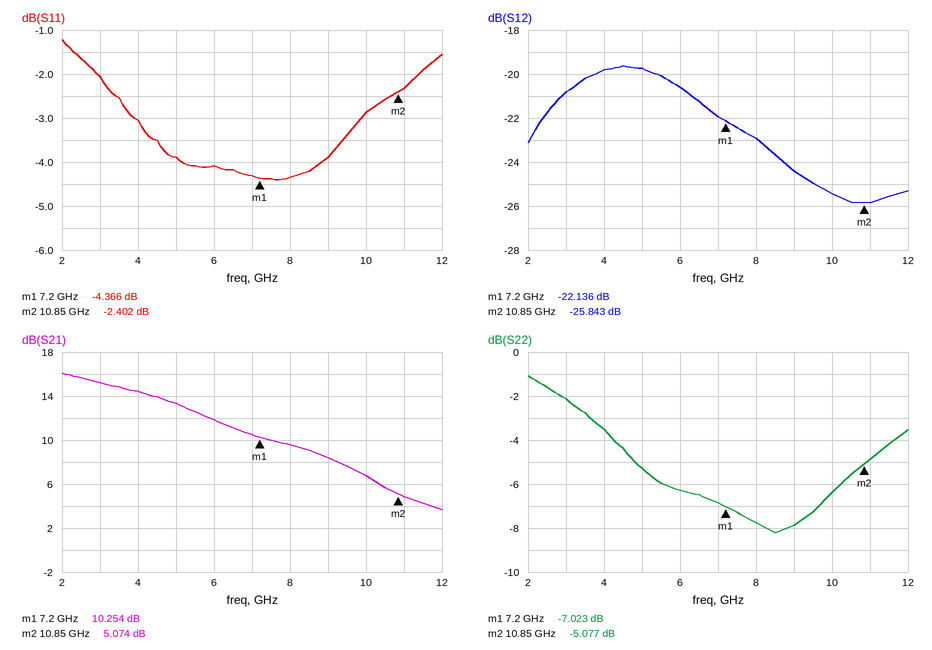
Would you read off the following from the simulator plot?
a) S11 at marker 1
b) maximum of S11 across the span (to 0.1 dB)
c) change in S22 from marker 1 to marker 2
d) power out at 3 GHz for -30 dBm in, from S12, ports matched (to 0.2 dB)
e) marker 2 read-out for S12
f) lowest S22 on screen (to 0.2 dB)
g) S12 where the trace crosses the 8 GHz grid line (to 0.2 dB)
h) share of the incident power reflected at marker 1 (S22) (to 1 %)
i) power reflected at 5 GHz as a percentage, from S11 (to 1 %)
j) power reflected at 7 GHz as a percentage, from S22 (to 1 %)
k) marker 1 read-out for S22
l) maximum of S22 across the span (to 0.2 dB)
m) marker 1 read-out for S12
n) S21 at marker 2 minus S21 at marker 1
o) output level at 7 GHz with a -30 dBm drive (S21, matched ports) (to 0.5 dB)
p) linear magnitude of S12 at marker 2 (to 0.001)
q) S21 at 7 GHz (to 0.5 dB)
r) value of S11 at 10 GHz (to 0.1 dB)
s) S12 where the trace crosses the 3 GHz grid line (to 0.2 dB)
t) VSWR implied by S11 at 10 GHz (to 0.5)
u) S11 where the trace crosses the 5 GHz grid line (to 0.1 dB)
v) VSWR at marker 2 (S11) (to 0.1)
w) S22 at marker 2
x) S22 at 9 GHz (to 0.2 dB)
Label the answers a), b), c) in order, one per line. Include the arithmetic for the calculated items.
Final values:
a) -4.366 dB
b) -1.2 dB
c) -5.077 − (-7.023) = 1.946 dB
d) -30 dBm + (-20.8 dB) = -50.8 dBm
e) -25.843 dB
f) -8.2 dB
g) -23.0 dB
h) 10^(-7.023/10) ≈ 20 %
i) 10^(-3.9/10) ≈ 41 %
j) 10^(-6.8/10) ≈ 21 %
k) -7.023 dB
l) -1.0 dB
m) -22.136 dB
n) 5.074 − (10.254) = -5.180 dB
o) -30 dBm + (10.5 dB) = -19.5 dBm
p) 10^(-25.843/20) ≈ 0.051
q) 10.5 dB
r) -2.9 dB
s) -20.8 dB
t) |Γ| = 10^(-2.9/20) = 0.7161; VSWR = (1 + 0.7161)/(1 − 0.7161) ≈ 6.0
u) -3.9 dB
v) (1 + 0.7584)/(1 − 0.7584) ≈ 7.3
w) -5.077 dB
x) -7.8 dB
